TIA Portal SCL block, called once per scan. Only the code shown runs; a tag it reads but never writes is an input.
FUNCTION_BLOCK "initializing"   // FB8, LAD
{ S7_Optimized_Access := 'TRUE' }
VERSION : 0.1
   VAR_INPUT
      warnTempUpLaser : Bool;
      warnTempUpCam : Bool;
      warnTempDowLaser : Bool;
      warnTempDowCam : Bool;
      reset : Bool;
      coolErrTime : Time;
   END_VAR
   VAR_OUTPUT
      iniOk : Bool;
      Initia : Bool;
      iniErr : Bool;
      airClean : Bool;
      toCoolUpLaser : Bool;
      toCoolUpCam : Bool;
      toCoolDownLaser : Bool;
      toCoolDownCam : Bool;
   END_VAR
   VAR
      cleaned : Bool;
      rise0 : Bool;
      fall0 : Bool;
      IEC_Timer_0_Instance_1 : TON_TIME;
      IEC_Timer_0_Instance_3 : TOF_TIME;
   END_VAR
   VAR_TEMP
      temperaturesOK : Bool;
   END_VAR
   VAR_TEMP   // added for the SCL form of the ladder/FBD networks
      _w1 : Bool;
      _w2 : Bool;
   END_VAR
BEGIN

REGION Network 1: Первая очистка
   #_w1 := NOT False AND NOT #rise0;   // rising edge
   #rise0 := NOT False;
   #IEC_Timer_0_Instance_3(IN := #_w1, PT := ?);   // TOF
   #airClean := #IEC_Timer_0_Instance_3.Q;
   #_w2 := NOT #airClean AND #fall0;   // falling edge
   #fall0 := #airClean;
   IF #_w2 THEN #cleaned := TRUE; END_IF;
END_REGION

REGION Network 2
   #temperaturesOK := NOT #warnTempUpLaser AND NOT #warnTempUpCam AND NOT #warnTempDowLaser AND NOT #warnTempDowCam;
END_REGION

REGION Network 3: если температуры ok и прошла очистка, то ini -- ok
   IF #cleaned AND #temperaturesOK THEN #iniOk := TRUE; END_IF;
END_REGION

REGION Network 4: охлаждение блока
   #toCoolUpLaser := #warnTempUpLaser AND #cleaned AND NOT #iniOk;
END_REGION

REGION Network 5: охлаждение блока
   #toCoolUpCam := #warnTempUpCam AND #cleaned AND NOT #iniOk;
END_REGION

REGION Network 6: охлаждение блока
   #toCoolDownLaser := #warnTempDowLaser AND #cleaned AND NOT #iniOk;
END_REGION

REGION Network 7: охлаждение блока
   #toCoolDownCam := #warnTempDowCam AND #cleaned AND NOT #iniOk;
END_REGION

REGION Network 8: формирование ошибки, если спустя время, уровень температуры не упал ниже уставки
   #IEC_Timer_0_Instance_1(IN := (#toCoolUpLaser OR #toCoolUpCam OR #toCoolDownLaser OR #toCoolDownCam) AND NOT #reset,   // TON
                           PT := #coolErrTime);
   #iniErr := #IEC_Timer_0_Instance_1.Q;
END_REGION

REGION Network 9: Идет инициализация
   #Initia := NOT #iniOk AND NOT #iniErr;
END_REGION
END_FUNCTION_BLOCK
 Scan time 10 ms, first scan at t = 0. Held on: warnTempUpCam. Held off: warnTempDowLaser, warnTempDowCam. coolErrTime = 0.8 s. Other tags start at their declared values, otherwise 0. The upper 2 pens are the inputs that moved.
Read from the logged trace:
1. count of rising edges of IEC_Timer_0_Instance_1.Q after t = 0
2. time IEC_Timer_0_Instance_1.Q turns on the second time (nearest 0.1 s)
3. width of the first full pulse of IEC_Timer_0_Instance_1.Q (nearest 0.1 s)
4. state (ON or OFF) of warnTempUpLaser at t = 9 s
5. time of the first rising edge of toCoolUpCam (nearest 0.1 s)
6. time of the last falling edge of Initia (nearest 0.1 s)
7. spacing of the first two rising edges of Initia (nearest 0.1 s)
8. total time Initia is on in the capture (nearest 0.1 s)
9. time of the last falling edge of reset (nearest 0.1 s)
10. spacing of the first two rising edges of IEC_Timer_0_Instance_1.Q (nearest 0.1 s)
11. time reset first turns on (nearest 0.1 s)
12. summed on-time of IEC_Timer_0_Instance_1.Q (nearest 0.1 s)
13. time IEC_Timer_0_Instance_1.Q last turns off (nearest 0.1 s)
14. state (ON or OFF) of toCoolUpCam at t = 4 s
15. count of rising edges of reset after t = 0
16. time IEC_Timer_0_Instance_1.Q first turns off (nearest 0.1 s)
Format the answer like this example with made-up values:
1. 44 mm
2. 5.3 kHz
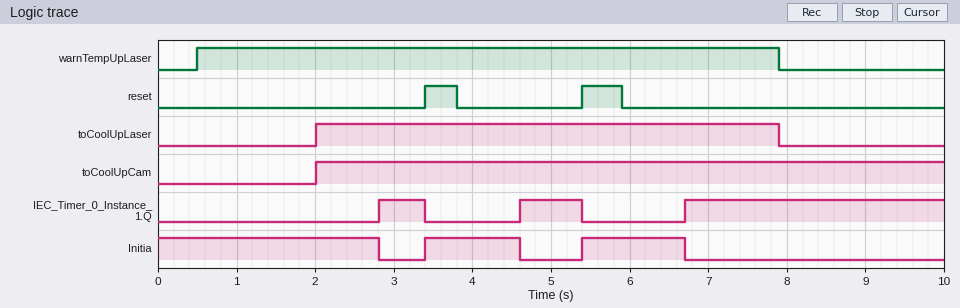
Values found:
1. 3
2. 4.6 s
3. 0.6 s
4. OFF
5. 2.0 s
6. 6.7 s
7. 2.0 s
8. 5.3 s
9. 5.9 s
10. 1.8 s
11. 3.4 s
12. 4.7 s
13. 5.4 s
14. ON
15. 2
16. 3.4 s
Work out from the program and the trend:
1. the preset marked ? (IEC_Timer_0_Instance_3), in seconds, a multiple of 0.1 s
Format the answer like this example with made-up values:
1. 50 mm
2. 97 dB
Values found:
1. 2.0 s
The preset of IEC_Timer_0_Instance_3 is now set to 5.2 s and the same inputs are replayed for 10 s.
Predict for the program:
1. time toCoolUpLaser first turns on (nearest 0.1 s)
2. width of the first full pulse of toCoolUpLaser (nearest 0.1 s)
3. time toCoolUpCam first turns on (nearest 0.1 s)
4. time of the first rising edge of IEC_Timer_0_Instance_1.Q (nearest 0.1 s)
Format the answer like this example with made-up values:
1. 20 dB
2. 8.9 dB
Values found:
1. 5.2 s
2. 2.7 s
3. 5.2 s
4. 6.7 s
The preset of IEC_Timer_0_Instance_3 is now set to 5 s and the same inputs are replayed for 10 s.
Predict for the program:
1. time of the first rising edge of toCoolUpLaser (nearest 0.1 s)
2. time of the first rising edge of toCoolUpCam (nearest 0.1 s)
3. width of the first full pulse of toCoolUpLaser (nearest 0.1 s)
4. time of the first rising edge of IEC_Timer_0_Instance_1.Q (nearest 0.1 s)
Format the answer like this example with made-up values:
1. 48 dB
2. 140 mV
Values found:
1. 5.0 s
2. 5.0 s
3. 2.9 s
4. 6.7 s
